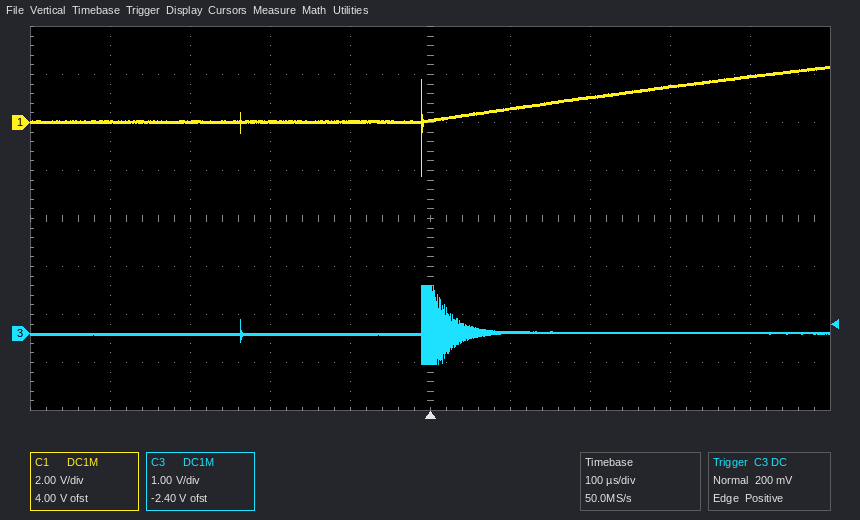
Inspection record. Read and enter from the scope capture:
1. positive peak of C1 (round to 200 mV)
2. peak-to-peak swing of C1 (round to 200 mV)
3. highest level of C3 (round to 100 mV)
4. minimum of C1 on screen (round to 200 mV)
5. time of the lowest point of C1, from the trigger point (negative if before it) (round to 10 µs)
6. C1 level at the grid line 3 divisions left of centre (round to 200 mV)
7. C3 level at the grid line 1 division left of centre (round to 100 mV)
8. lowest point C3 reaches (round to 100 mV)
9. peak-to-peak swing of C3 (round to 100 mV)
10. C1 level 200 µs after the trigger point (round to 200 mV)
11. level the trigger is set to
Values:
2.4 V
4.6 V
1.0 V
-2.2 V
-10 µs
0.0 V
0.0 V
-600 mV
1.6 V
1.0 V
200 mV
